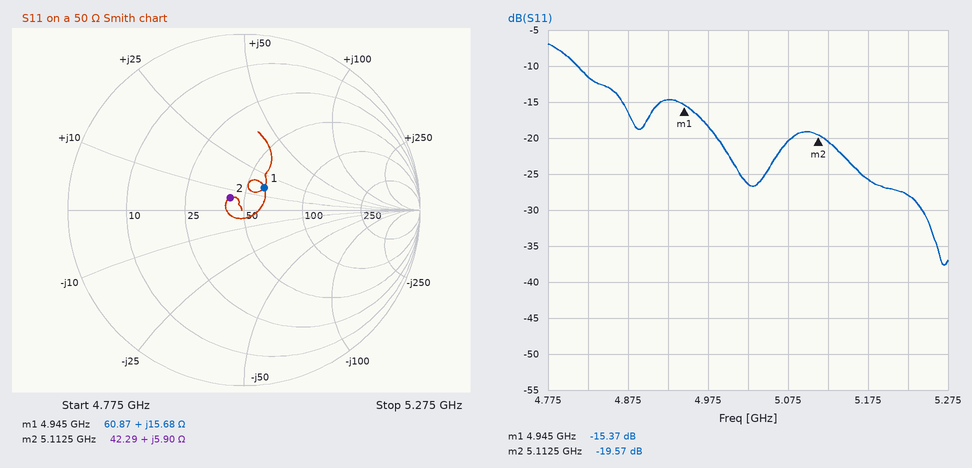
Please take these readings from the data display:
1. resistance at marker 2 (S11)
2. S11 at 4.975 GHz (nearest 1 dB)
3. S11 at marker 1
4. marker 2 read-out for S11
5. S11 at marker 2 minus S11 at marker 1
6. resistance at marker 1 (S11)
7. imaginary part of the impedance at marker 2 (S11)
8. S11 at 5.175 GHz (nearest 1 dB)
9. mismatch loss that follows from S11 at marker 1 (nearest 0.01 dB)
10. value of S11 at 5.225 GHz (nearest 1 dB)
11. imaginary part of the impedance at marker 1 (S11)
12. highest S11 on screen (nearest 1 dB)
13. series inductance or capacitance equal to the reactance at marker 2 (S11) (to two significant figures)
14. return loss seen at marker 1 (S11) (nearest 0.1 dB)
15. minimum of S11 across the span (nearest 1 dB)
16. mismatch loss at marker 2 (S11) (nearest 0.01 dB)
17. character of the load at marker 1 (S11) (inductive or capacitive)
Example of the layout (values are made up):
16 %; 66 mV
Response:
42.29 Ω; -18 dB; -15.37 dB; -19.57 dB; -4.20 dB; 60.87 Ω; +5.90 Ω; -26 dB; 0.13 dB; -28 dB; +15.68 Ω; -7 dB; 180 pH; 15.4 dB; -38 dB; 0.05 dB; inductive
